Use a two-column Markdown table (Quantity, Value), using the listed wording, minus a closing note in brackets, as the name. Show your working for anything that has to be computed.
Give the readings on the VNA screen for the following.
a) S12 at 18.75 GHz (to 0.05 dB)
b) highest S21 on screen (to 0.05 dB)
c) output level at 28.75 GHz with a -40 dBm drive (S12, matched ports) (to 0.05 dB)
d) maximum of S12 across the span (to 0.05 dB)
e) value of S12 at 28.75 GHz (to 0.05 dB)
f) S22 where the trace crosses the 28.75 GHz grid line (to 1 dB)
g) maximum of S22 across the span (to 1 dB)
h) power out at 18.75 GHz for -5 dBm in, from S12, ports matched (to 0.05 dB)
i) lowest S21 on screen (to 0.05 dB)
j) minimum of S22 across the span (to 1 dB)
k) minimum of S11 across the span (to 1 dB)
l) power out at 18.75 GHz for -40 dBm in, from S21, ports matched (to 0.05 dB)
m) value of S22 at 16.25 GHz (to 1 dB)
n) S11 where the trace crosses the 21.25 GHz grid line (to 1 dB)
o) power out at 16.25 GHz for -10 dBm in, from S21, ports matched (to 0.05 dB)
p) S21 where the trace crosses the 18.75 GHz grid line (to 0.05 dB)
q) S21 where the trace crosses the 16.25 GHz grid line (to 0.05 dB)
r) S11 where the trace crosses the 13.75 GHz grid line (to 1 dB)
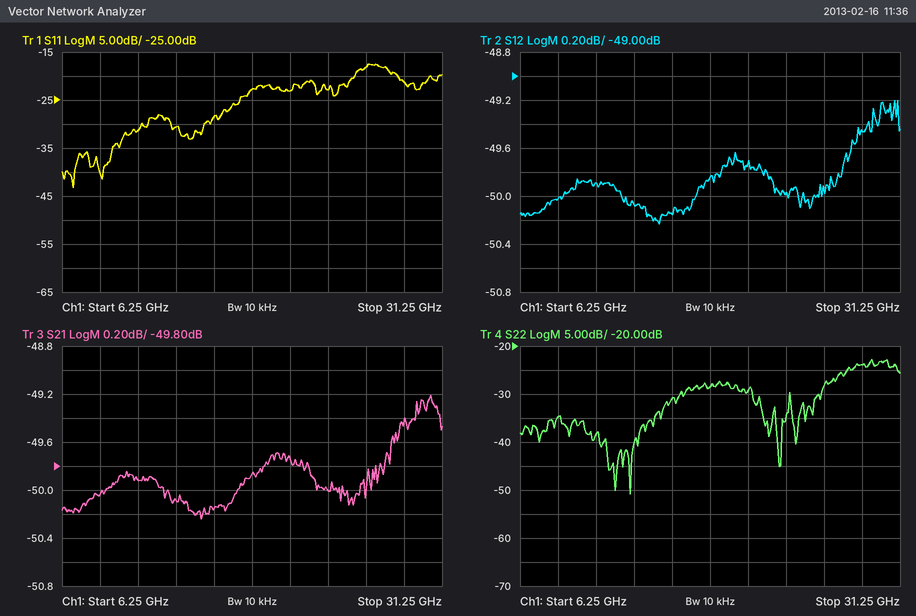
| Quantity | Value |
|---|---|
| S12 at 18.75 GHz | -49.85 dB |
| highest S21 on screen | -49.20 dB |
| output level at 28.75 GHz with a -40 dBm drive (S12, matched ports) | -40 dBm + (-49.45 dB) = -89.45 dBm |
| maximum of S12 across the span | -49.20 dB |
| value of S12 at 28.75 GHz | -49.45 dB |
| S22 where the trace crosses the 28.75 GHz grid line | -24 dB |
| maximum of S22 across the span | -23 dB |
| power out at 18.75 GHz for -5 dBm in, from S12, ports matched | -5 dBm + (-49.85 dB) = -54.85 dBm |
| lowest S21 on screen | -50.25 dB |
| minimum of S22 across the span | -51 dB |
| minimum of S11 across the span | -43 dB |
| power out at 18.75 GHz for -40 dBm in, from S21, ports matched | -40 dBm + (-49.85 dB) = -89.85 dBm |
| value of S22 at 16.25 GHz | -31 dB |
| S11 where the trace crosses the 21.25 GHz grid line | -23 dB |
| power out at 16.25 GHz for -10 dBm in, from S21, ports matched | -10 dBm + (-50.15 dB) = -60.15 dBm |
| S21 where the trace crosses the 18.75 GHz grid line | -49.85 dB |
| S21 where the trace crosses the 16.25 GHz grid line | -50.15 dB |
| S11 where the trace crosses the 13.75 GHz grid line | -31 dB |
